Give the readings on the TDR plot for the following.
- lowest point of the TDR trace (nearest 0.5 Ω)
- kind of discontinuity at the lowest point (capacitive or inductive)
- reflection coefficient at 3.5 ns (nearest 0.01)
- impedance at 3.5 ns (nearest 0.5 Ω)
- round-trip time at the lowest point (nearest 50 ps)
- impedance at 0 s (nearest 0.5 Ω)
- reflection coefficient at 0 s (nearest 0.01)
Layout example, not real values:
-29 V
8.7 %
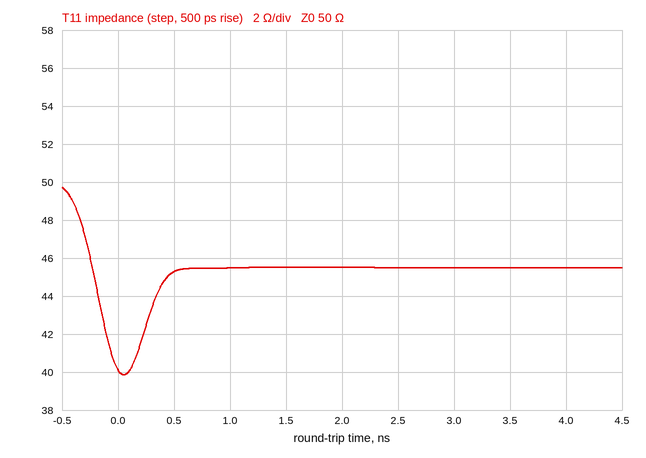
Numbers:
40.0 Ω
capacitive
-0.05
45.5 Ω
50 ps
40.0 Ω
-0.11
